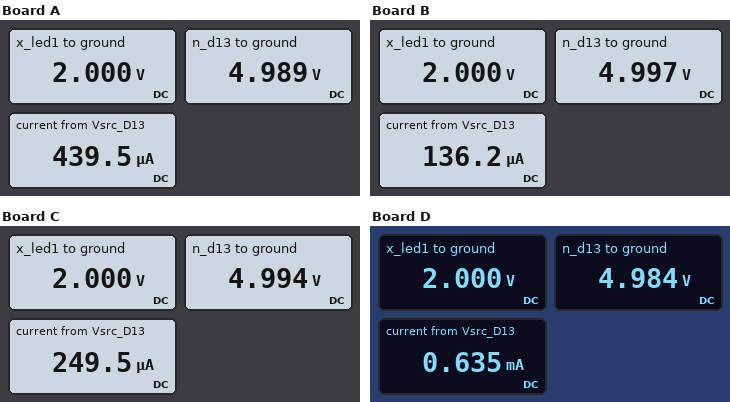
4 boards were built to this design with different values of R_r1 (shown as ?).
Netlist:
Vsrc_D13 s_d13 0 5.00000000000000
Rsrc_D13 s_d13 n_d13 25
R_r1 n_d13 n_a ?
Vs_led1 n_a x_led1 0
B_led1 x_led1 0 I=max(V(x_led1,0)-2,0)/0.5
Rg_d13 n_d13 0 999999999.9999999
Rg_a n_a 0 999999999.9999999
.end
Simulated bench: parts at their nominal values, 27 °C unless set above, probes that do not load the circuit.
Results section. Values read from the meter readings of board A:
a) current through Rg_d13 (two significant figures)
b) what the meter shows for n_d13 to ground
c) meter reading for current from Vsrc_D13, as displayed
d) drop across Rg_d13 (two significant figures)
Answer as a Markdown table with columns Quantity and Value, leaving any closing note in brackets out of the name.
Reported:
| Quantity | Value |
|---|---|
| current through Rg_d13 | 5.0 nA |
| what the meter shows for n_d13 to ground | 4.989 V |
| meter reading for current from Vsrc_D13, as displayed | 439.5 µA |
| drop across Rg_d13 | 5.0 V |
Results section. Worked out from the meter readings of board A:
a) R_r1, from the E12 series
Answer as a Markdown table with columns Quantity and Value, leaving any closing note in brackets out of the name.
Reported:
| Quantity | Value |
|---|---|
| R_r1, from the E12 series | 6.8 kΩ |
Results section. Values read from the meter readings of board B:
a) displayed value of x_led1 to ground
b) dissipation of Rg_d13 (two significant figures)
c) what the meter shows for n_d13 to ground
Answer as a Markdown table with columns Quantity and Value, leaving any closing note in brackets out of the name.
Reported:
| Quantity | Value |
|---|---|
| displayed value of x_led1 to ground | 2.000 V |
| dissipation of Rg_d13 | 25 nW |
| what the meter shows for n_d13 to ground | 4.997 V |
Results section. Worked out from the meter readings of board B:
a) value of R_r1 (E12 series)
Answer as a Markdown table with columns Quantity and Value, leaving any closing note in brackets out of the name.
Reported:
| Quantity | Value |
|---|---|
| value of R_r1 | 22 kΩ |
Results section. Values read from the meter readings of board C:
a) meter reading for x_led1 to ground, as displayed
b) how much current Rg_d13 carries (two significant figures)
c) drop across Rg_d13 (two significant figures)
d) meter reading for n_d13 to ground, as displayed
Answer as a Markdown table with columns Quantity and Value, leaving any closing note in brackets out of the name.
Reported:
| Quantity | Value |
|---|---|
| meter reading for x_led1 to ground, as displayed | 2.000 V |
| how much current Rg_d13 carries | 5.0 nA |
| drop across Rg_d13 | 5.0 V |
| meter reading for n_d13 to ground, as displayed | 4.994 V |
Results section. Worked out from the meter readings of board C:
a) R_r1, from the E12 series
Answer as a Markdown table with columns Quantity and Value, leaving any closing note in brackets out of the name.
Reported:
| Quantity | Value |
|---|---|
| R_r1, from the E12 series | 12 kΩ |
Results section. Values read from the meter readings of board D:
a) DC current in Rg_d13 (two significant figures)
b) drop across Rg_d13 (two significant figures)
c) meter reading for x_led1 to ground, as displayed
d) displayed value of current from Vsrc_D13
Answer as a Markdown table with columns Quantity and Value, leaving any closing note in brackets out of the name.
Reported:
| Quantity | Value |
|---|---|
| DC current in Rg_d13 | 5.0 nA |
| drop across Rg_d13 | 5.0 V |
| meter reading for x_led1 to ground, as displayed | 2.000 V |
| displayed value of current from Vsrc_D13 | 0.635 mA |
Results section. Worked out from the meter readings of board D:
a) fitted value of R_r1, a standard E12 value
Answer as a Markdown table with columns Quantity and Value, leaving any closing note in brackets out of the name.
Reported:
| Quantity | Value |
|---|---|
| fitted value of R_r1, a standard E12 value | 4.7 kΩ |
